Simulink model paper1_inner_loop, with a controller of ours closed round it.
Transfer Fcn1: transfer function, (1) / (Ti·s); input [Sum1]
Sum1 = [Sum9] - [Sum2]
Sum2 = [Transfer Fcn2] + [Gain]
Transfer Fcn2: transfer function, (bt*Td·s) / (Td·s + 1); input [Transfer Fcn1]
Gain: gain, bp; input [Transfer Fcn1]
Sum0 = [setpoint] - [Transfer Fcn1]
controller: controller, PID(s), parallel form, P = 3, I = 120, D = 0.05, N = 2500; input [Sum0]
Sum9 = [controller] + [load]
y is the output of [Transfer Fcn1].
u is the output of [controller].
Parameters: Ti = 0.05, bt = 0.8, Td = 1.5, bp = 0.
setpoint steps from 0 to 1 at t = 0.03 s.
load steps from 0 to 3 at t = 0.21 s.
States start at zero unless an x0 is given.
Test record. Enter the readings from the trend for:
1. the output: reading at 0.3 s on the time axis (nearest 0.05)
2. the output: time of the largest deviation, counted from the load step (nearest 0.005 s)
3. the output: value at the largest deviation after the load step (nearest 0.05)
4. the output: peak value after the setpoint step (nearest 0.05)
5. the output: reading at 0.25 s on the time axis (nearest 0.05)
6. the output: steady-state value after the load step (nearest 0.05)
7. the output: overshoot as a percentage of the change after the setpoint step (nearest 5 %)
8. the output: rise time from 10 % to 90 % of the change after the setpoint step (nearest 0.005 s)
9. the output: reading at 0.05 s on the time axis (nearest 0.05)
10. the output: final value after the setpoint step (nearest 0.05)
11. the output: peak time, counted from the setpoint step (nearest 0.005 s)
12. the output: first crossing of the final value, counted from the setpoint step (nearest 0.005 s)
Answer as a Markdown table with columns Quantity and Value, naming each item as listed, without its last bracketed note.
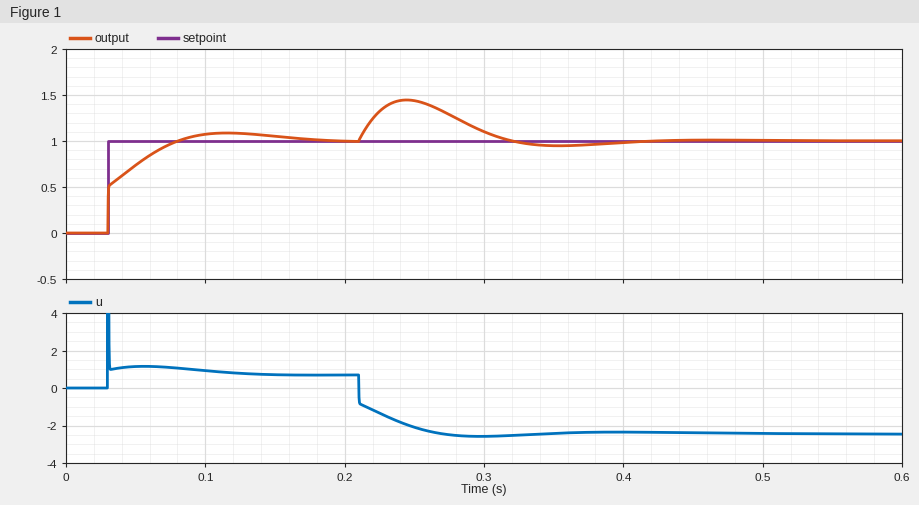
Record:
| Quantity | Value |
|---|---|
| the output: reading at 0.3 s on the time axis | 1.10 |
| the output: time of the largest deviation, counted from the load step | 0.035 s |
| the output: value at the largest deviation after the load step | 1.45 |
| the output: peak value after the setpoint step | 1.10 |
| the output: reading at 0.25 s on the time axis | 1.45 |
| the output: steady-state value after the load step | 1.00 |
| the output: overshoot as a percentage of the change after the setpoint step | 10 % |
| the output: rise time from 10 % to 90 % of the change after the setpoint step | 0.035 s |
| the output: reading at 0.05 s on the time axis | 0.75 |
| the output: final value after the setpoint step | 1.00 |
| the output: peak time, counted from the setpoint step | 0.085 s |
| the output: first crossing of the final value, counted from the setpoint step | 0.050 s |
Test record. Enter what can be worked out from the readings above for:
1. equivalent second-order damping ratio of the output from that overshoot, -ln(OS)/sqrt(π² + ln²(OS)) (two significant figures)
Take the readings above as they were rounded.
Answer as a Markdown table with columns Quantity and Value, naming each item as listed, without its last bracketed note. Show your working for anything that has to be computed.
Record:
| Quantity | Value |
|---|---|
| equivalent second-order damping ratio of the output from that overshoot, -ln(OS)/sqrt(π² + ln²(OS)) | ln(0.1) = -2.303; 2.303 / sqrt(9.870 + 5.302) = 0.59 |
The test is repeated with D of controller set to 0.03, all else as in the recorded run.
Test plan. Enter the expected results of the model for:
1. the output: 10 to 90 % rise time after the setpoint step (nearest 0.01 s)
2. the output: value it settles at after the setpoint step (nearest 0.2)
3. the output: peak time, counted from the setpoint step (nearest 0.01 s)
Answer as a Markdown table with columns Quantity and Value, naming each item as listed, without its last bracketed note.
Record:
| Quantity | Value |
|---|---|
| the output: 10 to 90 % rise time after the setpoint step | 0.03 s |
| the output: value it settles at after the setpoint step | 1.0 |
| the output: peak time, counted from the setpoint step | 0.07 s |
